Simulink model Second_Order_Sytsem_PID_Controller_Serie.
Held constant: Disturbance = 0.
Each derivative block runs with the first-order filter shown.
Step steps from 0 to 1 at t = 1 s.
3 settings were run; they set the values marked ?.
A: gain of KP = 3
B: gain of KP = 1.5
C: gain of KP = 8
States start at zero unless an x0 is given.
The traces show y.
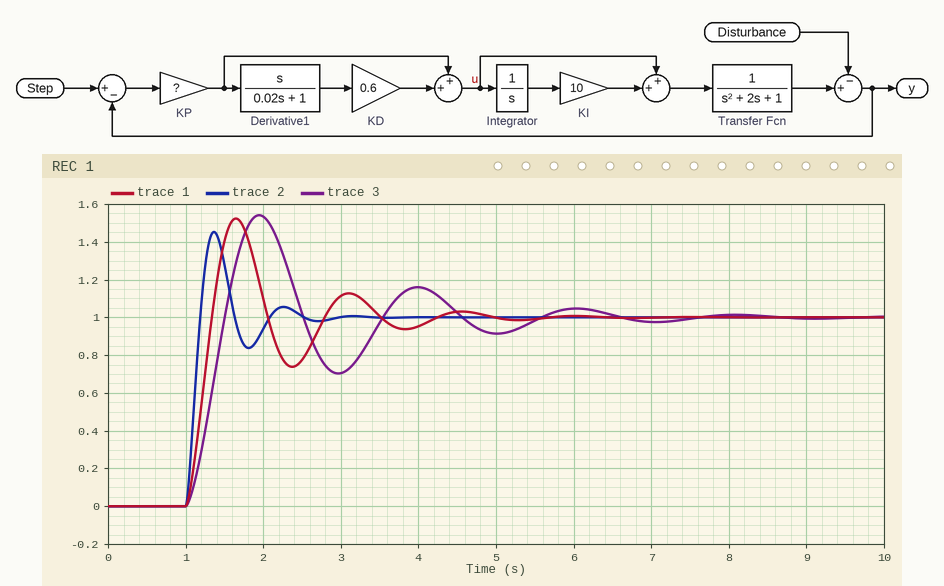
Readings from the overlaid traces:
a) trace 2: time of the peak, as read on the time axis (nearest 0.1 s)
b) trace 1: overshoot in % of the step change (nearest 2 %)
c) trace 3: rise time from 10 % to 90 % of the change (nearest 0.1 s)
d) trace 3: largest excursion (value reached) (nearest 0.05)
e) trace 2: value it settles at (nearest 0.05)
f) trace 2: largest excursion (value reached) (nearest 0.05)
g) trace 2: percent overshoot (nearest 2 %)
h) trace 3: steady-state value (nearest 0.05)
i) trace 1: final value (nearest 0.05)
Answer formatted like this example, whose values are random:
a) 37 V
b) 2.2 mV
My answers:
a) 1.4 s
b) 52 %
c) 0.4 s
d) 1.55
e) 1.00
f) 1.45
g) 46 %
h) 1.00
i) 1.00
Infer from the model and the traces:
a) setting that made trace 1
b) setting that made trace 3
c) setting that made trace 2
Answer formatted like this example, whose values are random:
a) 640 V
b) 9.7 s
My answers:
a) A
b) B
c) C
